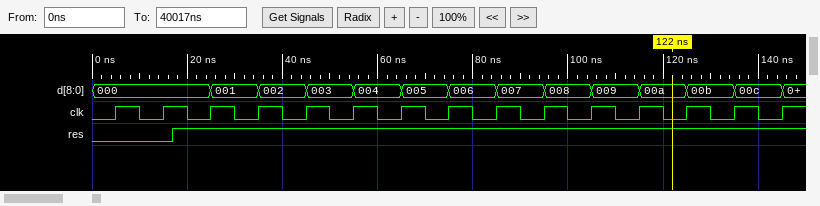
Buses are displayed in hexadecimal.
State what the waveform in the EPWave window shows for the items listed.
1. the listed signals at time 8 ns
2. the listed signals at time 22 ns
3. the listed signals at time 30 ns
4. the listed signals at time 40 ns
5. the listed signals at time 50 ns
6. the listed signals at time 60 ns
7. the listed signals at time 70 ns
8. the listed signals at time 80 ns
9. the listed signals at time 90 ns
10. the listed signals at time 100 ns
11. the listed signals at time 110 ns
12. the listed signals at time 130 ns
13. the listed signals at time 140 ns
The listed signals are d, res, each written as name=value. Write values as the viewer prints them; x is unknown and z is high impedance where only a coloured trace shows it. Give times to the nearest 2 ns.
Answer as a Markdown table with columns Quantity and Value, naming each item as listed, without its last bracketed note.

| Quantity | Value |
|---|---|
| the listed signals at time 8 ns | d=000, res=0 |
| the listed signals at time 22 ns | d=000, res=1 |
| the listed signals at time 30 ns | d=001, res=1 |
| the listed signals at time 40 ns | d=002, res=1 |
| the listed signals at time 50 ns | d=003, res=1 |
| the listed signals at time 60 ns | d=004, res=1 |
| the listed signals at time 70 ns | d=005, res=1 |
| the listed signals at time 80 ns | d=006, res=1 |
| the listed signals at time 90 ns | d=007, res=1 |
| the listed signals at time 100 ns | d=008, res=1 |
| the listed signals at time 110 ns | d=009, res=1 |
| the listed signals at time 130 ns | d=00b, res=1 |
| the listed signals at time 140 ns | d=00c, res=1 |
